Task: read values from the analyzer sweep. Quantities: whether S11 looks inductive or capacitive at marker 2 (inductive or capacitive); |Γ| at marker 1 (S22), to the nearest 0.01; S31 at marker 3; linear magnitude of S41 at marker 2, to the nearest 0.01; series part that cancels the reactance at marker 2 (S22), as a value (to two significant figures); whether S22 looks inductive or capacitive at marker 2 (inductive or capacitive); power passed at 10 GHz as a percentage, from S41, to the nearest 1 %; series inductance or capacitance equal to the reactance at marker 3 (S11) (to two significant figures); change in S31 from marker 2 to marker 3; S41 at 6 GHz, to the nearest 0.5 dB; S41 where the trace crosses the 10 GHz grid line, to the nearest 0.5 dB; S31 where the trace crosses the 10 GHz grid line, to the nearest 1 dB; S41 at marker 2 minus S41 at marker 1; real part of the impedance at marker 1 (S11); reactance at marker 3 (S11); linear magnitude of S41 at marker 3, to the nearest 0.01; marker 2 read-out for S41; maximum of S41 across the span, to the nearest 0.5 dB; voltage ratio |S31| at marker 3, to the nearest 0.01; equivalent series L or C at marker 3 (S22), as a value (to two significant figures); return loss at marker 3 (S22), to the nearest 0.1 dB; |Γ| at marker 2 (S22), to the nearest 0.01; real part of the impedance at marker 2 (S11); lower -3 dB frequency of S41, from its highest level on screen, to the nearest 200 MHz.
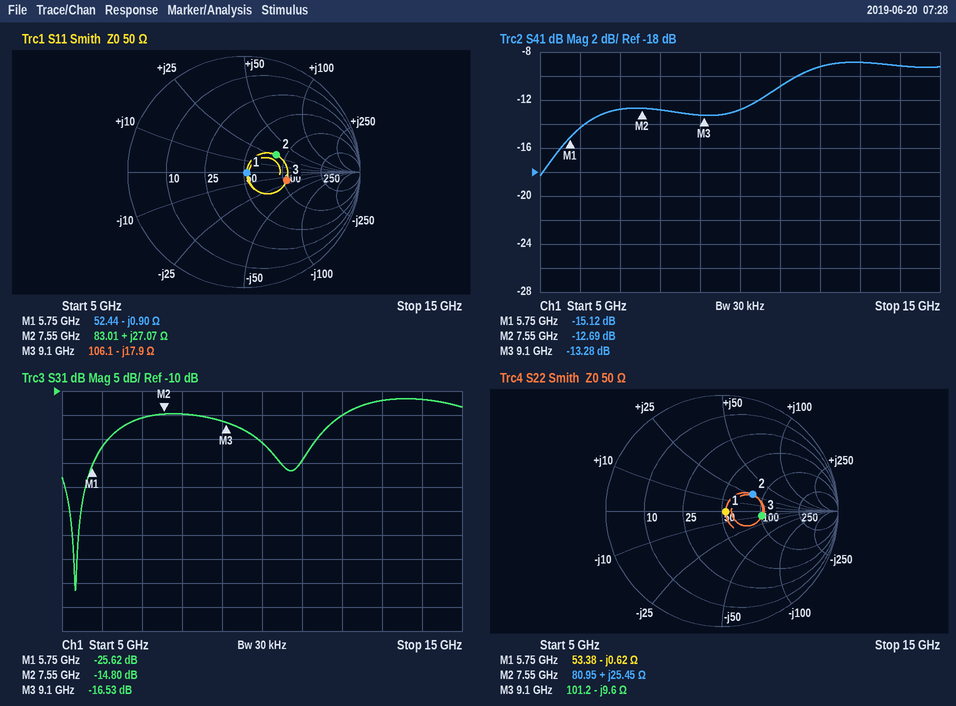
inductive
0.03
-16.53 dB
0.23
830 fF
inductive
5 %
980 fF
-1.73 dB
-14.5 dB
-13.0 dB
-21 dB
2.43 dB
52.44 Ω
-17.9 Ω
0.22
-12.69 dB
-9.0 dB
0.15
1.8 pF
9.3 dB
0.30
83.01 Ω
10.6 GHz
